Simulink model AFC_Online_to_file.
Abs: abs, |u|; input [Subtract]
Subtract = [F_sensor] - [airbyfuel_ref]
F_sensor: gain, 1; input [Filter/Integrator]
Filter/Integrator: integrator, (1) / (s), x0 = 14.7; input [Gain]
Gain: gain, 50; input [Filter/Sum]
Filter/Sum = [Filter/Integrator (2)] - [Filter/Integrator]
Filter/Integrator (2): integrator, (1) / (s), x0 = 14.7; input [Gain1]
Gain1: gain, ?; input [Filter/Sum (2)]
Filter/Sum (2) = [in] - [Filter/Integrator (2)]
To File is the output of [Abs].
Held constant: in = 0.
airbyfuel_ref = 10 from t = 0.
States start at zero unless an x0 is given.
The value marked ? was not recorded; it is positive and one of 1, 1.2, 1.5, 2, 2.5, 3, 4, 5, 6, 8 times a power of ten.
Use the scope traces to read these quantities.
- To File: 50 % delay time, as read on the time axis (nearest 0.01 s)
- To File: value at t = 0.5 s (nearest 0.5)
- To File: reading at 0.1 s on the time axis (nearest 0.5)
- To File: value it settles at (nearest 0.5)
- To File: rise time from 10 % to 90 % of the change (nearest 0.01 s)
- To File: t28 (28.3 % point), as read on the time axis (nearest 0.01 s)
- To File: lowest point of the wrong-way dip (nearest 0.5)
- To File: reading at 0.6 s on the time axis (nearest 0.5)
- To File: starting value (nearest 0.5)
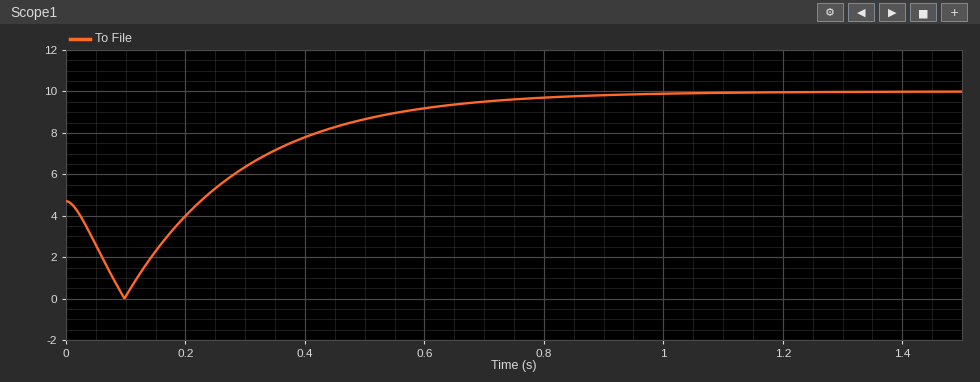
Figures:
0.36 s
8.5
0.0
10.0
0.44 s
0.29 s
0.0
9.0
4.5
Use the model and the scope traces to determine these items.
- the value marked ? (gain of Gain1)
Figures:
5
